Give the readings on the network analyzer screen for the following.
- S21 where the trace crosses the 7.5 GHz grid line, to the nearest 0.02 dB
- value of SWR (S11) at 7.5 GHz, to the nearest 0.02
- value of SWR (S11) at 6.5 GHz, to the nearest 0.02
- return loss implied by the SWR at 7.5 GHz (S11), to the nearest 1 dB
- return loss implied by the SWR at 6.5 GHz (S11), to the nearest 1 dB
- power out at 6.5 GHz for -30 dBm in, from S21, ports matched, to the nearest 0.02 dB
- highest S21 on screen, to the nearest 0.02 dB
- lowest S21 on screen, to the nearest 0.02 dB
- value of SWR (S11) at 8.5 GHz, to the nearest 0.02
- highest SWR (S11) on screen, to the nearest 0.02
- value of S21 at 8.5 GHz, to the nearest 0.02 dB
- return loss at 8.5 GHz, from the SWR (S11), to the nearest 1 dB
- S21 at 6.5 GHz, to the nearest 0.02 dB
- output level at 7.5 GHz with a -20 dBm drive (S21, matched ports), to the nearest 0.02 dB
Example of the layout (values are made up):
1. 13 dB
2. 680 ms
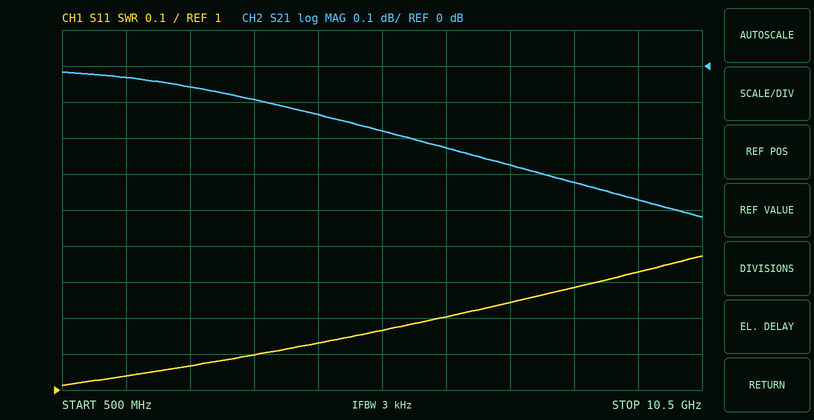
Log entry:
1. -0.28 dB
2. 1.24
3. 1.20
4. 19 dB
5. 21 dB
6. -30.22 dBm
7. -0.02 dB
8. -0.42 dB
9. 1.28
10. 1.38
11. -0.32 dB
12. 18 dB
13. -0.22 dB
14. -20.28 dBm
